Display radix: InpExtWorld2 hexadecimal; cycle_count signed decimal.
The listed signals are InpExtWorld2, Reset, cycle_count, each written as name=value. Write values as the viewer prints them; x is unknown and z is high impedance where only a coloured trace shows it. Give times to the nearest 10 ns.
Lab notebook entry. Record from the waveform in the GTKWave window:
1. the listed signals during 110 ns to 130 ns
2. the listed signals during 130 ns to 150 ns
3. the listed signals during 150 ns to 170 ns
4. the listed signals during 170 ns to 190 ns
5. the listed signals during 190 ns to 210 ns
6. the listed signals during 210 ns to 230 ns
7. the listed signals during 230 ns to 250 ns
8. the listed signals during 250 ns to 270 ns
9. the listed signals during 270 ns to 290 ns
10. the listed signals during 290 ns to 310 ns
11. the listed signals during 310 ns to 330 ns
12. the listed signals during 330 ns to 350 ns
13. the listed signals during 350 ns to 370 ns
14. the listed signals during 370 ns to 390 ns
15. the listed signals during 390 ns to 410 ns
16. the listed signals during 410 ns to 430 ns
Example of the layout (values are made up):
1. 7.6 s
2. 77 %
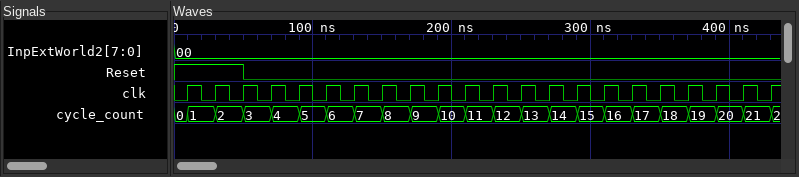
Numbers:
1. InpExtWorld2=00, Reset=0, cycle_count=6
2. InpExtWorld2=00, Reset=0, cycle_count=7
3. InpExtWorld2=00, Reset=0, cycle_count=8
4. InpExtWorld2=00, Reset=0, cycle_count=9
5. InpExtWorld2=00, Reset=0, cycle_count=10
6. InpExtWorld2=00, Reset=0, cycle_count=11
7. InpExtWorld2=00, Reset=0, cycle_count=12
8. InpExtWorld2=00, Reset=0, cycle_count=13
9. InpExtWorld2=00, Reset=0, cycle_count=14
10. InpExtWorld2=00, Reset=0, cycle_count=15
11. InpExtWorld2=00, Reset=0, cycle_count=16
12. InpExtWorld2=00, Reset=0, cycle_count=17
13. InpExtWorld2=00, Reset=0, cycle_count=18
14. InpExtWorld2=00, Reset=0, cycle_count=19
15. InpExtWorld2=00, Reset=0, cycle_count=20
16. InpExtWorld2=00, Reset=0, cycle_count=21
